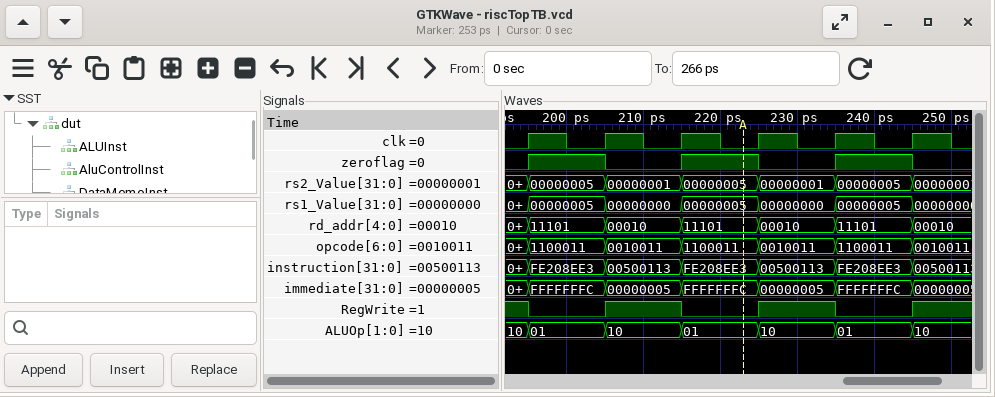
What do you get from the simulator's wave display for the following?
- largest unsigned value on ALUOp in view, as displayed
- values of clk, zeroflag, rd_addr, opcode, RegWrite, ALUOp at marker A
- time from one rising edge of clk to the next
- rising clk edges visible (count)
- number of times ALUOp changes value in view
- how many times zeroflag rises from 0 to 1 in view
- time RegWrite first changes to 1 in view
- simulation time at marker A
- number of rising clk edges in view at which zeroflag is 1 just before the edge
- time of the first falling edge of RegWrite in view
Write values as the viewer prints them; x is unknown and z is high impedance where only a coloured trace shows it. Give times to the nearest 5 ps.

10
clk=0, zeroflag=1, rd_addr=11101, opcode=1100011, RegWrite=0, ALUOp=01
10 ps
6
6
3
205 ps
225 ps
3
195 ps
